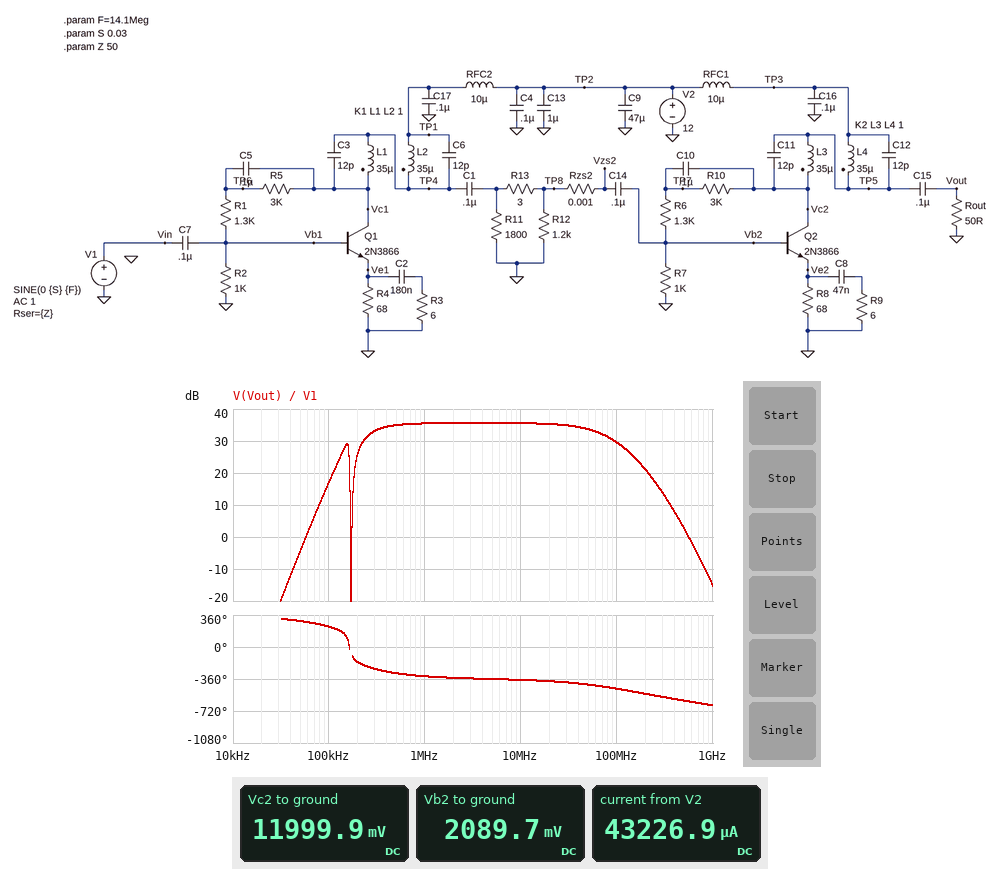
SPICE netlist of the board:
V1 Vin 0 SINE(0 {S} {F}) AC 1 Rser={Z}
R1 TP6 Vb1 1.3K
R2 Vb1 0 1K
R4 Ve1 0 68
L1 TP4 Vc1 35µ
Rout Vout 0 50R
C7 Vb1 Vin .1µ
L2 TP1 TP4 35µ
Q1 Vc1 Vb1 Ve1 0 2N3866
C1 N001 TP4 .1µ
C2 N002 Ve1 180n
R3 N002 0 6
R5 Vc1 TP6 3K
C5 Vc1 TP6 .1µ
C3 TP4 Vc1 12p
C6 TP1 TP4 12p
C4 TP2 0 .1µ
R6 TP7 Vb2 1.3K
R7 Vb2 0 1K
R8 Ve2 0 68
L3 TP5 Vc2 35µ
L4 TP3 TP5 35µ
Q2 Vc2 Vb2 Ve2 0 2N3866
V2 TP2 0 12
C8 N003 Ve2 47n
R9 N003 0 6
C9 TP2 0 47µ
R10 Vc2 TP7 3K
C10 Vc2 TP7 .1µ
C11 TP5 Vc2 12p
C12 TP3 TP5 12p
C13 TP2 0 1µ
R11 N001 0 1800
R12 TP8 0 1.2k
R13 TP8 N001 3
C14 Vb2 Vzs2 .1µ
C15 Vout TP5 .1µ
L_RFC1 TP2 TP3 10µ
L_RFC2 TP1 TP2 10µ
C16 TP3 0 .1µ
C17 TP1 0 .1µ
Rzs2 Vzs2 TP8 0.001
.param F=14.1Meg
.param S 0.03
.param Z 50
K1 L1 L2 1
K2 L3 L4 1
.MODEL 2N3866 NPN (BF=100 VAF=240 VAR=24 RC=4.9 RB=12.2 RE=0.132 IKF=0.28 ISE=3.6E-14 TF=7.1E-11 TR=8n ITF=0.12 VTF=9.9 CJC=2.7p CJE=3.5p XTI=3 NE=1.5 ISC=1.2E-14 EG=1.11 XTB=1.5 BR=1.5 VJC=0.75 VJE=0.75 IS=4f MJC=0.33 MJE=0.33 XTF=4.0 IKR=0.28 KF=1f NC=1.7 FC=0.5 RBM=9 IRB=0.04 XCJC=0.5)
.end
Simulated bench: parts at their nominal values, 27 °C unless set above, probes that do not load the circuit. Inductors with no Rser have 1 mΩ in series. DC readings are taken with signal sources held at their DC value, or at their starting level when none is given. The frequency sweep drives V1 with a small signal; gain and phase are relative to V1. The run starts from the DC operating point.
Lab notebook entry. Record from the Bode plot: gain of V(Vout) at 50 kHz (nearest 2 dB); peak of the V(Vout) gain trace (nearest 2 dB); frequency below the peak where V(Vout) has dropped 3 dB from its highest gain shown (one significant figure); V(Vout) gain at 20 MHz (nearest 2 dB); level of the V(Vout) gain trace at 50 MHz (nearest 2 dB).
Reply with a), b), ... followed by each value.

a) -4 dB
b) 36 dB
c) 300 kHz
d) 36 dB
e) 34 dB
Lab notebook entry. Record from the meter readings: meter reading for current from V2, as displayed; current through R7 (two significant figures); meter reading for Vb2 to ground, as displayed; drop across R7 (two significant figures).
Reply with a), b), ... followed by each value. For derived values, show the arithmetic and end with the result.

a) 43226.9 µA
b) (2.09 V) / 1 kΩ = 2.1 mA
c) 2089.7 mV
d) 2.09 V = 2.1 V
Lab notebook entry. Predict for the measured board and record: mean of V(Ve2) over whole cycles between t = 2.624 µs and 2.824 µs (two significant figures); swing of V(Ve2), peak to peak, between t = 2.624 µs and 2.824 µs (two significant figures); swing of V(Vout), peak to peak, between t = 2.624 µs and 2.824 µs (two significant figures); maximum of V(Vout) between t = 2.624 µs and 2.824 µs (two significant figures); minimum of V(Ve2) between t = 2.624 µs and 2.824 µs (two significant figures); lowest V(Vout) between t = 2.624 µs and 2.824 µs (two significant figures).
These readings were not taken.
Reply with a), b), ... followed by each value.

a) 1.3 V
b) 220 mV
c) 3.3 V
d) 1.6 V
e) 1.2 V
f) -1.7 V
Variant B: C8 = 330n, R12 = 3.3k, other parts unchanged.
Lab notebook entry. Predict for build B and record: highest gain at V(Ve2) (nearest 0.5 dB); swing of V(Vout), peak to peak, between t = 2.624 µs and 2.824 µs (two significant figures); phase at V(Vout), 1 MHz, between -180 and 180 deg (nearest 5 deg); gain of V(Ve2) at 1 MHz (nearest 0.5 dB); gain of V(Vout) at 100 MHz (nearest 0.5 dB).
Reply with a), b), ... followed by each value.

a) 15.5 dB
b) 3.4 V
c) 20 deg
d) 12.0 dB
e) 29.5 dB
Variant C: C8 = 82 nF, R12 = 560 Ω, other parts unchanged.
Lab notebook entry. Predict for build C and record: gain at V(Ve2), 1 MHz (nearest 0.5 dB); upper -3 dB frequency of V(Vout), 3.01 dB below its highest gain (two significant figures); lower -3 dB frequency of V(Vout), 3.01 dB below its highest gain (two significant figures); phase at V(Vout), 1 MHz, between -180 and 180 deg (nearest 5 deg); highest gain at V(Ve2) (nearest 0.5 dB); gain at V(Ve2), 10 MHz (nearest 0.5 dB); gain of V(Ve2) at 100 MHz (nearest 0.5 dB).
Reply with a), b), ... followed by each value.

a) 12.0 dB
b) 65 MHz
c) 230 kHz
d) 25 deg
e) 18.5 dB
f) 11.5 dB
g) 7.5 dB
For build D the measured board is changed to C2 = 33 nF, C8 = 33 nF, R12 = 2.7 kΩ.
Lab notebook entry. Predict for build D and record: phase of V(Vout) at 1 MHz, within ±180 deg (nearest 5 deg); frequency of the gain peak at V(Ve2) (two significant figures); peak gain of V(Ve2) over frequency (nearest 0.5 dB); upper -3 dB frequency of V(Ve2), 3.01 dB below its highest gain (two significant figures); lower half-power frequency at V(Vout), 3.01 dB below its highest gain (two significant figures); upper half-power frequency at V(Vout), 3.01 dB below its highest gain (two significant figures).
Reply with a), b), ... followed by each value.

a) 45 deg
b) 320 kHz
c) 17.0 dB
d) 670 kHz
e) 390 kHz
f) 65 MHz
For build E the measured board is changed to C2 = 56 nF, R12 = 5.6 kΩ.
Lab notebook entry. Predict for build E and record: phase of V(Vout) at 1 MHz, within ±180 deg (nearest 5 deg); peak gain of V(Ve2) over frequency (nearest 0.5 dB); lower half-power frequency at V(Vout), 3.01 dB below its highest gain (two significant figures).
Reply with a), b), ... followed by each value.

a) 35 deg
b) 18.5 dB
c) 270 kHz
